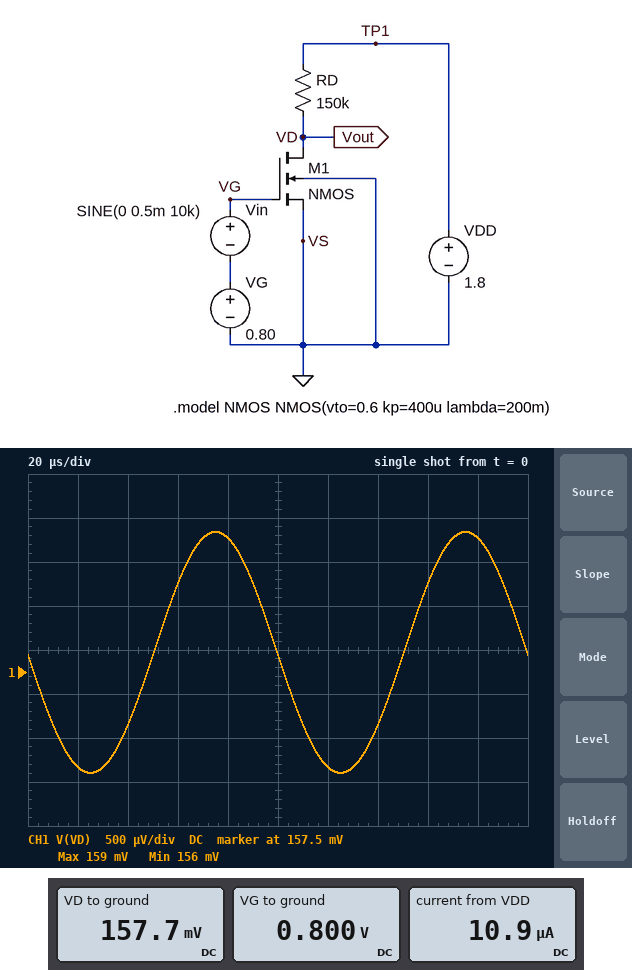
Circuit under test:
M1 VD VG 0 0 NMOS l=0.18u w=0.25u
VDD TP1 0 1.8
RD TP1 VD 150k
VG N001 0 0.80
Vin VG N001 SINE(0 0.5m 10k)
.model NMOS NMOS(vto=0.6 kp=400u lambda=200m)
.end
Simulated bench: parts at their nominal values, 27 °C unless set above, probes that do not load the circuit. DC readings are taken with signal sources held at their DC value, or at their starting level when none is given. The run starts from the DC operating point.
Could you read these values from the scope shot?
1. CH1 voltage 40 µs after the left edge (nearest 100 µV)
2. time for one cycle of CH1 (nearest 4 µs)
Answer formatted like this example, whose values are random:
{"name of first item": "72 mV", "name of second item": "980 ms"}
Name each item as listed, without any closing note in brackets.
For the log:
{"CH1 voltage 40 µs after the left edge": "156.9 mV", "time for one cycle of CH1": "100 µs"}
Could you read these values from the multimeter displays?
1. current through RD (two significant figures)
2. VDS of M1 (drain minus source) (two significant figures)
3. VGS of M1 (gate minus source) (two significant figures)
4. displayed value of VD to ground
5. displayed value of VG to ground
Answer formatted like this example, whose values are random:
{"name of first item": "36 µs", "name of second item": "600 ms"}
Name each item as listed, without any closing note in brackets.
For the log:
{"current through RD": "11 µA", "VDS of M1 (drain minus source)": "160 mV", "VGS of M1 (gate minus source)": "800 mV", "displayed value of VD to ground": "157.7 mV", "displayed value of VG to ground": "0.800 V"}
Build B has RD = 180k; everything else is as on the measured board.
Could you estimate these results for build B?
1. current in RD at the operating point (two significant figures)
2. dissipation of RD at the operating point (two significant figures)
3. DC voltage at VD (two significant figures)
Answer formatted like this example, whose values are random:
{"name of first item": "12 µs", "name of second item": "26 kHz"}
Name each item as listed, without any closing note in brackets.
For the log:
{"current in RD at the operating point": "9.4 µA", "dissipation of RD at the operating point": "16 µW", "DC voltage at VD": "120 mV"}
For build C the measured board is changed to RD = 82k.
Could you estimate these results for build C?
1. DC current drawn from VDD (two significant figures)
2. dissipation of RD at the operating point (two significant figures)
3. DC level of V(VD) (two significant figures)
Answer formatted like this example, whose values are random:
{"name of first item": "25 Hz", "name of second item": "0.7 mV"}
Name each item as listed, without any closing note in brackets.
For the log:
{"DC current drawn from VDD": "13 µA", "dissipation of RD at the operating point": "13 µW", "DC level of V(VD)": "750 mV"}
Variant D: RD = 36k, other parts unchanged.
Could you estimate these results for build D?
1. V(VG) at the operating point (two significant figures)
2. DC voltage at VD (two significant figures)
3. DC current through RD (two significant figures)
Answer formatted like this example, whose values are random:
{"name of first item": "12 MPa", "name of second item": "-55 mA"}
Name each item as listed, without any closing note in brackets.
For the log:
{"V(VG) at the operating point": "800 mV", "DC voltage at VD": "1.3 V", "DC current through RD": "14 µA"}
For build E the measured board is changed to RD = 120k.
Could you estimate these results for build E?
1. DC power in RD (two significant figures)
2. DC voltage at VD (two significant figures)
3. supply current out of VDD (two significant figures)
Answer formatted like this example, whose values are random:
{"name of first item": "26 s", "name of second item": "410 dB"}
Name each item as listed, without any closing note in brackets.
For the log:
{"DC power in RD": "17 µW", "DC voltage at VD": "370 mV", "supply current out of VDD": "12 µA"}
